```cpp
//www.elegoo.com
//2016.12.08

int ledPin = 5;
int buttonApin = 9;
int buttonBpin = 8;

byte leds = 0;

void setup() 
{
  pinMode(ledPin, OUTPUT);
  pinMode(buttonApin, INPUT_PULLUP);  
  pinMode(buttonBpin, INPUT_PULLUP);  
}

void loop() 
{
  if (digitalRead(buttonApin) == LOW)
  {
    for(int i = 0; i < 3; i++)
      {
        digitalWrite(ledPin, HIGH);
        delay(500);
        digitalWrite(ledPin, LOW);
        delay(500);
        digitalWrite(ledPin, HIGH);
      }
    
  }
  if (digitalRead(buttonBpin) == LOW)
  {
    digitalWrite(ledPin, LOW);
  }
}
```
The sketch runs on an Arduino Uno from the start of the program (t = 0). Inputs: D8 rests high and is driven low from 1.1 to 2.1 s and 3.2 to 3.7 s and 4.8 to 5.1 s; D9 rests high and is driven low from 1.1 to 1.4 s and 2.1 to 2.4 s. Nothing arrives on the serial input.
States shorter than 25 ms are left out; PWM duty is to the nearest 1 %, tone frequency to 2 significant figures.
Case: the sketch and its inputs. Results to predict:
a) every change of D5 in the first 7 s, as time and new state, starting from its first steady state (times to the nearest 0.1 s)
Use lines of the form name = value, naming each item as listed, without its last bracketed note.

every change of D5 in the first 7 s, as time and new state, starting from its first steady state = 0 s low; 1.1 s high; 1.6 s low; 2.1 s high; 2.6 s low; 3.1 s high; 3.6 s low; 4.1 s high; 4.8 s low
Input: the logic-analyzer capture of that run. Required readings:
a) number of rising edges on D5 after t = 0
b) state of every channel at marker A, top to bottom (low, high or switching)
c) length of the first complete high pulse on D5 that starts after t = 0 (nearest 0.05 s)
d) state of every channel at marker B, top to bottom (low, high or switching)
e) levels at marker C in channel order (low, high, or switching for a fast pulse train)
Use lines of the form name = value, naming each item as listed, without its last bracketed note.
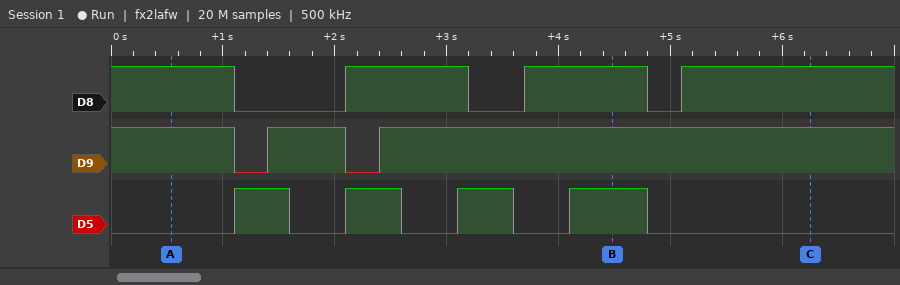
number of rising edges on D5 after t = 0 = 4
state of every channel at marker A, top to bottom = D8 high, D9 high, D5 low
length of the first complete high pulse on D5 that starts after t = 0 = 0.50 s
state of every channel at marker B, top to bottom = D8 high, D9 high, D5 high
levels at marker C in channel order = D8 high, D9 high, D5 low
